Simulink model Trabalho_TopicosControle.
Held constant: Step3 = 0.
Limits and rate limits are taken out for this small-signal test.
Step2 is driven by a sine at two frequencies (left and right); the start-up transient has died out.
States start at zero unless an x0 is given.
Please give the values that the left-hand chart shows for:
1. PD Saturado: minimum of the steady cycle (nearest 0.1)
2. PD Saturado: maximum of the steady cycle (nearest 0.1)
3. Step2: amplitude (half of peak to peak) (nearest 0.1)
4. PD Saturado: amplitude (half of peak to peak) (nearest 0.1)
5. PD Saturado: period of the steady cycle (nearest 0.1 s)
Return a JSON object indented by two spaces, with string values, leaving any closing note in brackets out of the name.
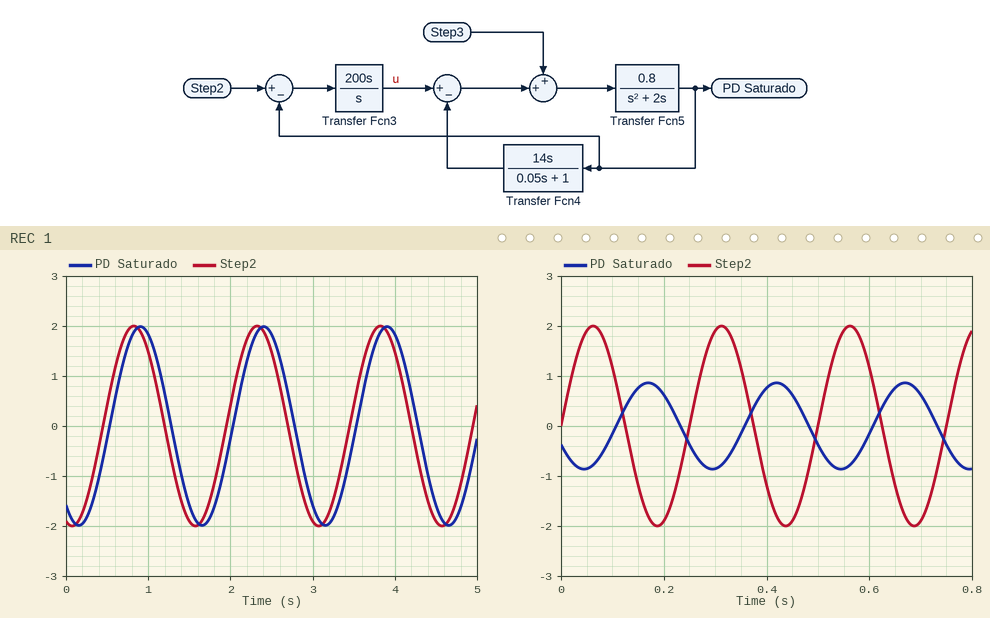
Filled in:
{
  "PD Saturado: minimum of the steady cycle": "-2.0",
  "PD Saturado: maximum of the steady cycle": "2.0",
  "Step2: amplitude (half of peak to peak)": "2.0",
  "PD Saturado: amplitude (half of peak to peak)": "2.0",
  "PD Saturado: period of the steady cycle": "1.5 s"
}
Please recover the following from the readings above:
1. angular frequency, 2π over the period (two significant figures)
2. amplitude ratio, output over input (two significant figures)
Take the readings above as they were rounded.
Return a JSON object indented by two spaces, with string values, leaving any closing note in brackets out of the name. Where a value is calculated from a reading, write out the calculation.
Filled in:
{
  "angular frequency, 2π over the period": "2π / 1.5 = 4.2 rad/s",
  "amplitude ratio, output over input": "2 / 2 = 1.0"
}
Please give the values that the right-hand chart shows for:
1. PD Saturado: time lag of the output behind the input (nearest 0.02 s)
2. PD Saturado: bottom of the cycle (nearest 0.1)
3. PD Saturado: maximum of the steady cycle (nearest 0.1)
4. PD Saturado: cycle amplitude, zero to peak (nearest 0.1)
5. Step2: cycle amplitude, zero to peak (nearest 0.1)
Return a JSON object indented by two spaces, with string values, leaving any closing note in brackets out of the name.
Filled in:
{
  "PD Saturado: time lag of the output behind the input": "0.10 s",
  "PD Saturado: bottom of the cycle": "-0.9",
  "PD Saturado: maximum of the steady cycle": "0.9",
  "PD Saturado: cycle amplitude, zero to peak": "0.9",
  "Step2: cycle amplitude, zero to peak": "2.0"
}
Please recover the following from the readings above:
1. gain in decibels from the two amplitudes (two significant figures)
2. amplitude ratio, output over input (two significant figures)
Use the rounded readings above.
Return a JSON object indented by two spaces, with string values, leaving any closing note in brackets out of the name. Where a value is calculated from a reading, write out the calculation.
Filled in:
{
  "gain in decibels from the two amplitudes": "20 log10(0.9 / 2) = -6.9 dB",
  "amplitude ratio, output over input": "0.9 / 2 = 0.45"
}
